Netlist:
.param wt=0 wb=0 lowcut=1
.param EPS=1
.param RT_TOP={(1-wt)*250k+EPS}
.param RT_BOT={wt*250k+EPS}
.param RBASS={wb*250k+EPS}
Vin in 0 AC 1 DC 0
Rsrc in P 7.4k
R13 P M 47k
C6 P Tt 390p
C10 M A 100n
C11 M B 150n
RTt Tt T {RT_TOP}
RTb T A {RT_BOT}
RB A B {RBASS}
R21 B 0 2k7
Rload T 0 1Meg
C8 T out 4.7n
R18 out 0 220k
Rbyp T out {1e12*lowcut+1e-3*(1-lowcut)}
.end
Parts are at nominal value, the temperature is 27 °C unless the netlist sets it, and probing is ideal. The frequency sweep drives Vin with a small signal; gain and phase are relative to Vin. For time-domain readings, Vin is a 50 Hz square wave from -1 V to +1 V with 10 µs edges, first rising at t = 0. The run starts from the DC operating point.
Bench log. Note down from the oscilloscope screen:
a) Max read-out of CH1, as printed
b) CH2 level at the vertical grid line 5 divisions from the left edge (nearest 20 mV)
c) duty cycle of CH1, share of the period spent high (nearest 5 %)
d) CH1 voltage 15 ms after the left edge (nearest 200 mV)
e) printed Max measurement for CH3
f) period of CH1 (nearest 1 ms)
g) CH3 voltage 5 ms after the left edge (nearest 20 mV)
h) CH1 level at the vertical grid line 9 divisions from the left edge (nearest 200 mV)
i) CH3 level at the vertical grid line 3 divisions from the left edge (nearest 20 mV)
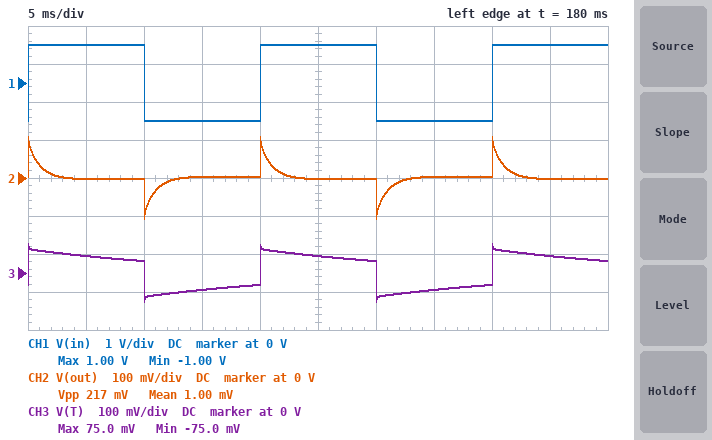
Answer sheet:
1.00 V
0 V
50 %
-1.0 V
75.0 mV
20 ms
40 mV
1.0 V
-40 mV
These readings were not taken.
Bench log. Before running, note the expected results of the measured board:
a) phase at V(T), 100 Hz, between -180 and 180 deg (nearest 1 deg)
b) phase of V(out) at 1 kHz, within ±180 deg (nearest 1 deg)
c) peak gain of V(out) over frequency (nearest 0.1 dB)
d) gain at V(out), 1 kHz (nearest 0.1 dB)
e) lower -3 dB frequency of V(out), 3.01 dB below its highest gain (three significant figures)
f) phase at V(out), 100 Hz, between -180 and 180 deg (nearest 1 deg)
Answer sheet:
7 deg
13 deg
-25.4 dB
-26.3 dB
211 Hz
64 deg
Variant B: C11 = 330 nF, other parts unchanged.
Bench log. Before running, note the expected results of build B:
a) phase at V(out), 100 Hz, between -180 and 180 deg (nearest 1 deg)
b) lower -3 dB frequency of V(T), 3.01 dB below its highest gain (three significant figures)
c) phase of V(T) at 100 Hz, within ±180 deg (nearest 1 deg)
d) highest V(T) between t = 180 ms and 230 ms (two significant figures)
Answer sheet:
61 deg
8.74 Hz
4 deg
69 mV
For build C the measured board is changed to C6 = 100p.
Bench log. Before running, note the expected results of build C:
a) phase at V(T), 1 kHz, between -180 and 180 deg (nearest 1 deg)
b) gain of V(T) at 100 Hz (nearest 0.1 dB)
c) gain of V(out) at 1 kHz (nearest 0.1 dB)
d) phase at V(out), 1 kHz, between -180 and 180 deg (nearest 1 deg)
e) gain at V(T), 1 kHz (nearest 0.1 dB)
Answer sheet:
2 deg
-26.6 dB
-26.7 dB
11 deg
-26.6 dB
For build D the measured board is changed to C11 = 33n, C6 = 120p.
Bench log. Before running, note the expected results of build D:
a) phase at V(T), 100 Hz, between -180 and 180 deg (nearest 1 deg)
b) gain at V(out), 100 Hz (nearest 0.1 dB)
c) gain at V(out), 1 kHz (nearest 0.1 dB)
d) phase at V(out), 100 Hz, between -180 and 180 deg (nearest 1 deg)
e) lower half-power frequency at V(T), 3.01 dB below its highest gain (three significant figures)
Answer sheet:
12 deg
-32.0 dB
-26.7 dB
69 deg
28.3 Hz
